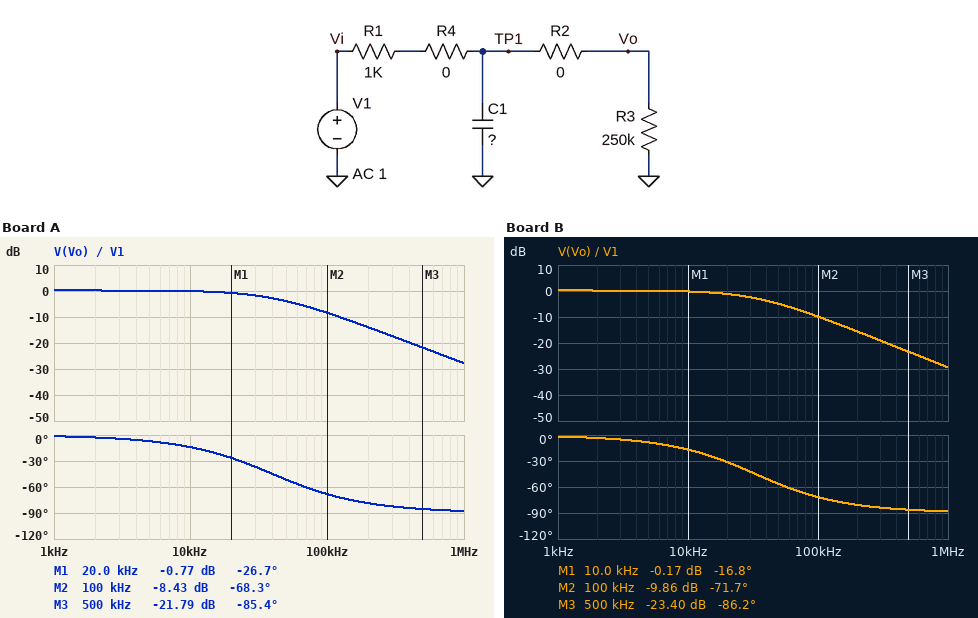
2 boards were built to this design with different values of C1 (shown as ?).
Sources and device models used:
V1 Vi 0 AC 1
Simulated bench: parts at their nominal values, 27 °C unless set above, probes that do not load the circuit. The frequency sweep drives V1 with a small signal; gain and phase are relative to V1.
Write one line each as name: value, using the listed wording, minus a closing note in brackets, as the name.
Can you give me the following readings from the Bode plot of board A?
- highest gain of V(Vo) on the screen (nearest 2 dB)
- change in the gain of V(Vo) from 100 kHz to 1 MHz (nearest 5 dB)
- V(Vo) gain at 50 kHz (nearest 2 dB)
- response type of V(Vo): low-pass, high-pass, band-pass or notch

highest gain of V(Vo) on the screen: 0 dB
change in the gain of V(Vo) from 100 kHz to 1 MHz: -20 dB
V(Vo) gain at 50 kHz: -4 dB
response type of V(Vo): low-pass, high-pass, band-pass or notch: low-pass
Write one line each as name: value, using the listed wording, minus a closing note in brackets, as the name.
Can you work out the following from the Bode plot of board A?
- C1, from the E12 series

C1, from the E12 series: 3.9 nF
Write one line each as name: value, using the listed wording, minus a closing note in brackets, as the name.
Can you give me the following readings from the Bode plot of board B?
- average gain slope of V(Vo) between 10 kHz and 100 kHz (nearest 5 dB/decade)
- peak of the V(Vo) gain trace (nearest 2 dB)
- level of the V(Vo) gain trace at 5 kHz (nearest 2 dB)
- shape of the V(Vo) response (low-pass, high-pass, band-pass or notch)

average gain slope of V(Vo) between 10 kHz and 100 kHz: -10 dB/decade
peak of the V(Vo) gain trace: 0 dB
level of the V(Vo) gain trace at 5 kHz: 0 dB
shape of the V(Vo) response: low-pass
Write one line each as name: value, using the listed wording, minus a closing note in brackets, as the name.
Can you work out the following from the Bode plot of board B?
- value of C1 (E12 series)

value of C1: 4.7 nF
